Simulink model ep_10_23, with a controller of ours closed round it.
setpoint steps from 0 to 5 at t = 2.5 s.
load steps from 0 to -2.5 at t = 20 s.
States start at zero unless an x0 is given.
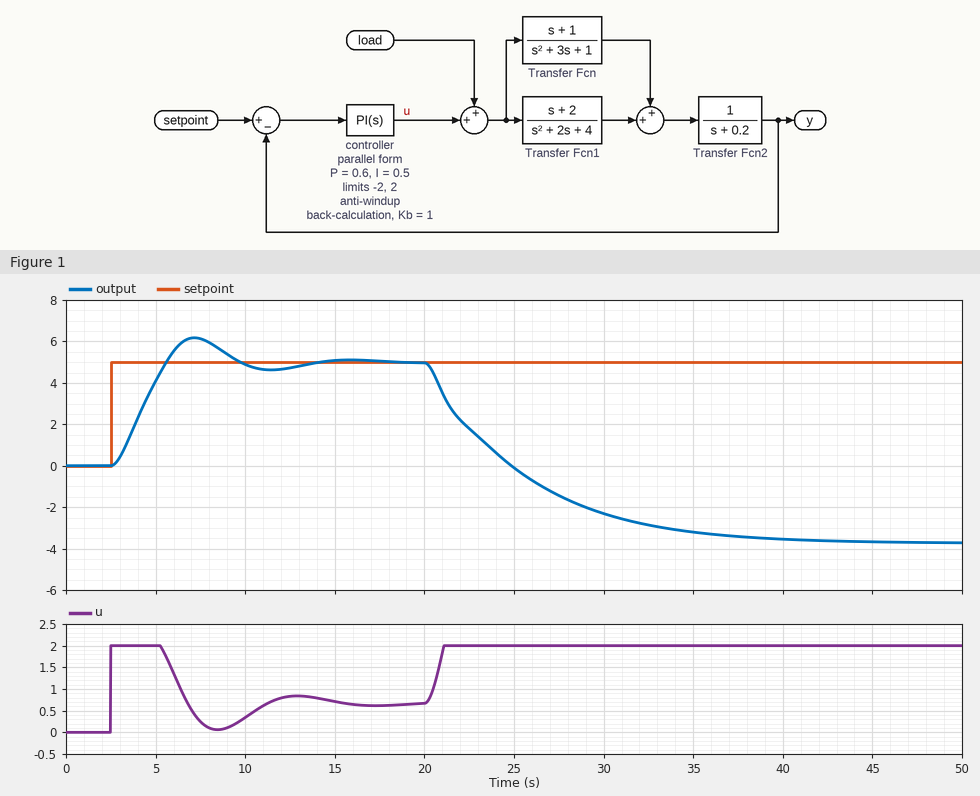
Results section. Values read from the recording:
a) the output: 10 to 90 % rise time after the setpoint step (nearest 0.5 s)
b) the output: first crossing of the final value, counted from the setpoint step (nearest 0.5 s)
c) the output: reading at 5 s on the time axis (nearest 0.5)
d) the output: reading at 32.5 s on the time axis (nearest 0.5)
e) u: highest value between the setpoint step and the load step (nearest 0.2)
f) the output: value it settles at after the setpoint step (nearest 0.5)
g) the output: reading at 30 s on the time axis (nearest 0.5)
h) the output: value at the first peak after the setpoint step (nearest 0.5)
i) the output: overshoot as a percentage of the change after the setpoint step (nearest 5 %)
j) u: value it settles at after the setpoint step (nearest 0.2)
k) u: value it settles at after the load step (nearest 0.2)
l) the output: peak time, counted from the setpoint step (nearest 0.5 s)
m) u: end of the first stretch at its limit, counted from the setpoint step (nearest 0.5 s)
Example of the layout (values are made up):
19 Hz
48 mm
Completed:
2.0 s
3.0 s
4.0
-3.0
2.0
5.0
-2.5
6.0
25 %
0.6
2.0
4.5 s
3.0 s
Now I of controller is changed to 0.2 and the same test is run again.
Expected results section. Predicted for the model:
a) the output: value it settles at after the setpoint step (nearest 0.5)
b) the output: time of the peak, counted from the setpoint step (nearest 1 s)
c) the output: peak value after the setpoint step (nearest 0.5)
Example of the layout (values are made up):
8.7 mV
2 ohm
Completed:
5.0
6 s
5.5
